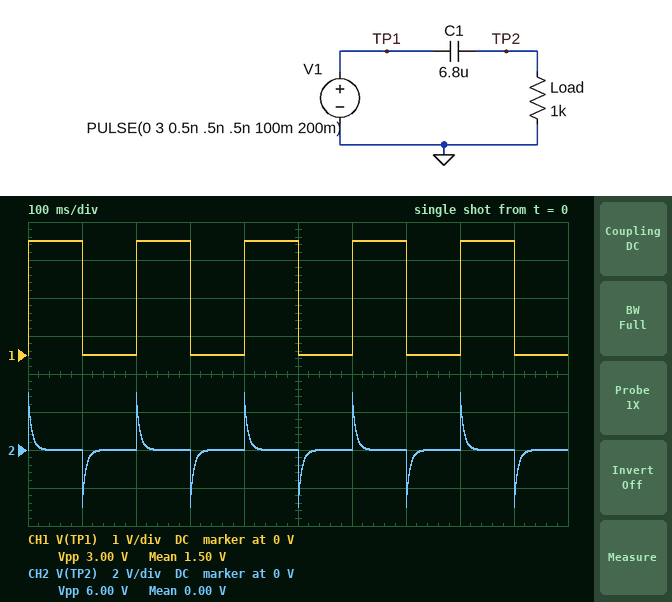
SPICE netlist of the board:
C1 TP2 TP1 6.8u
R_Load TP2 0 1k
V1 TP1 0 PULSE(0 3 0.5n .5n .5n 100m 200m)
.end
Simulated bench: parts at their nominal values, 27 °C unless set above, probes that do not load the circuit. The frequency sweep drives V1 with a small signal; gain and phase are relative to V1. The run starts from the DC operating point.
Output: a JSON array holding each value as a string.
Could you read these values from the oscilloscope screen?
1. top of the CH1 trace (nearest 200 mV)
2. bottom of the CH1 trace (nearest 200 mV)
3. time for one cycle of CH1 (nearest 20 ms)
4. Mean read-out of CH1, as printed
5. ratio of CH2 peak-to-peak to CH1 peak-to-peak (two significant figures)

["3.0 V", "0 V", "200 ms", "1.50 V", "2.0"]
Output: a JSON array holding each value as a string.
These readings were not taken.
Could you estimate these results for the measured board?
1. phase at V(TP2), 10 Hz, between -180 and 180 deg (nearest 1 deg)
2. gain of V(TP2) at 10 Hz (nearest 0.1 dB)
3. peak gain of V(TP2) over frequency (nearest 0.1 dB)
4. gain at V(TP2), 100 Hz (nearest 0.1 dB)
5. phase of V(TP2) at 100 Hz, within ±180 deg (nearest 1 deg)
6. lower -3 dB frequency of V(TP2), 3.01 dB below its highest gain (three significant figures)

["67 deg", "-8.1 dB", "0 dB", "-0.2 dB", "13 deg", "23.4 Hz"]
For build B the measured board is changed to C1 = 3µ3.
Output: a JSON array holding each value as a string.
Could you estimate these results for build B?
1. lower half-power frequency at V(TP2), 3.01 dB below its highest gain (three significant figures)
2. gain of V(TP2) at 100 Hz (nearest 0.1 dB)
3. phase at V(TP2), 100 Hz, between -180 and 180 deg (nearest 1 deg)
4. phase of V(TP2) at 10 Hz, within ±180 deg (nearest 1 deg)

["48.2 Hz", "-0.9 dB", "26 deg", "78 deg"]
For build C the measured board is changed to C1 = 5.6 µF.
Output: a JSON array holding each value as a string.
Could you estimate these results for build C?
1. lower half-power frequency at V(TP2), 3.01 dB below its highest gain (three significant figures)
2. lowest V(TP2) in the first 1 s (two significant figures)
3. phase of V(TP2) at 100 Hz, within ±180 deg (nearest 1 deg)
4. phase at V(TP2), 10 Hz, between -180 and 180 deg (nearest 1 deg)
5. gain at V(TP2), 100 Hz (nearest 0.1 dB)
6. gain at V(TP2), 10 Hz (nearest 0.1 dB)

["28.4 Hz", "-3.0 V", "16 deg", "71 deg", "-0.3 dB", "-9.6 dB"]
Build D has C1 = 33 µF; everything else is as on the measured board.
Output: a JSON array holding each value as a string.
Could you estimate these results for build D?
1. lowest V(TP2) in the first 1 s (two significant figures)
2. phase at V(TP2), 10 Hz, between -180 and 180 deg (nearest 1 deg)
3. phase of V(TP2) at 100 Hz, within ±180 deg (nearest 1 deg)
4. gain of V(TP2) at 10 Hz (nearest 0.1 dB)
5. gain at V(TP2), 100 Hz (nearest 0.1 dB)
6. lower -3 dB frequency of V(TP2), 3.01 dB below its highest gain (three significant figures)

["-2.9 V", "26 deg", "3 deg", "-0.9 dB", "0 dB", "4.82 Hz"]
